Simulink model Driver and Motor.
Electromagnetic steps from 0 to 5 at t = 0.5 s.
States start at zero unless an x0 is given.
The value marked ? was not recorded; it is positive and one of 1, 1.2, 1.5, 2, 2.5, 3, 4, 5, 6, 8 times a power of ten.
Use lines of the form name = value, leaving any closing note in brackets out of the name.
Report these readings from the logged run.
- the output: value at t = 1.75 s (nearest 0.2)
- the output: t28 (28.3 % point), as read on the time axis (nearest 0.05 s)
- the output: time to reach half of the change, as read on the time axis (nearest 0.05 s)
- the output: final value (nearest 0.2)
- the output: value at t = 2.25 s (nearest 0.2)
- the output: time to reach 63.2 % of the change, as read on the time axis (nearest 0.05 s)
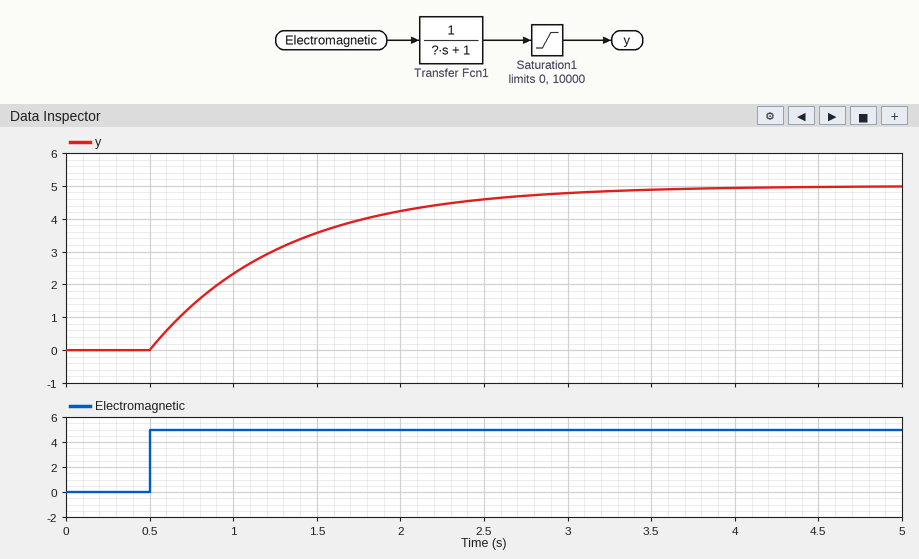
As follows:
the output: value at t = 1.75 s = 4.0
the output: t28 (28.3 % point), as read on the time axis = 0.75 s
the output: time to reach half of the change, as read on the time axis = 1.05 s
the output: final value = 5.0
the output: value at t = 2.25 s = 4.4
the output: time to reach 63.2 % of the change, as read on the time axis = 1.30 s
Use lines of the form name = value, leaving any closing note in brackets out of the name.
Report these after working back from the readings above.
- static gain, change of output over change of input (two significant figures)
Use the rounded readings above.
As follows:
static gain, change of output over change of input = 1.0
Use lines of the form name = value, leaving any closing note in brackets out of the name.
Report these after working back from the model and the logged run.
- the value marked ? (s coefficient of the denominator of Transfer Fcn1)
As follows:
the value marked ? = 0.8
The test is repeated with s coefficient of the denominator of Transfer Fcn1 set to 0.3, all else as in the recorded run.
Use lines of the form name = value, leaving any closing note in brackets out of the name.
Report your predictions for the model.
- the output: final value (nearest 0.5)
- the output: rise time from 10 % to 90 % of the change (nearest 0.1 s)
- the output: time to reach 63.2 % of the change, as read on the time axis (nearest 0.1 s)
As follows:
the output: final value = 5.0
the output: rise time from 10 % to 90 % of the change = 0.7 s
the output: time to reach 63.2 % of the change, as read on the time axis = 0.8 s
